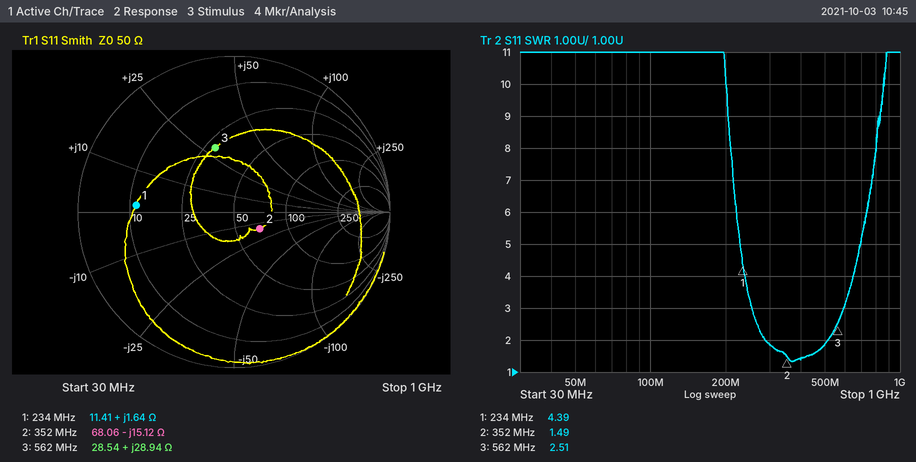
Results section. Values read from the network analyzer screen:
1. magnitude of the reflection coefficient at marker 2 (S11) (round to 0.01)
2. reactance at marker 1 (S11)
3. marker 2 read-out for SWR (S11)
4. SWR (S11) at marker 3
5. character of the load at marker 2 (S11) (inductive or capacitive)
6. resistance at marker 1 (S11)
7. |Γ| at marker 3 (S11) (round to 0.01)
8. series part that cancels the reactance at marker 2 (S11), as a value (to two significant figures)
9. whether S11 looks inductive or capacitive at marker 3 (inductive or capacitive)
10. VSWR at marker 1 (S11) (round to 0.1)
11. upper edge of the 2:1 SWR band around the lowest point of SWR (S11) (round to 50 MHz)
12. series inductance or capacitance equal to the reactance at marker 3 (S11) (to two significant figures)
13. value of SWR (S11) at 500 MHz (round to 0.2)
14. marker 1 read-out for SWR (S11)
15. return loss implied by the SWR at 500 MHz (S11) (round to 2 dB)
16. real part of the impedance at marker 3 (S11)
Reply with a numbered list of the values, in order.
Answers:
1. 0.20
2. +1.64 Ω
3. 1.49
4. 2.51
5. capacitive
6. 11.41 Ω
7. 0.43
8. 6.8 nH
9. inductive
10. 4.4
11. 500 MHz
12. 8.2 nH
13. 1.8
14. 4.39
15. 10 dB
16. 28.54 Ω
